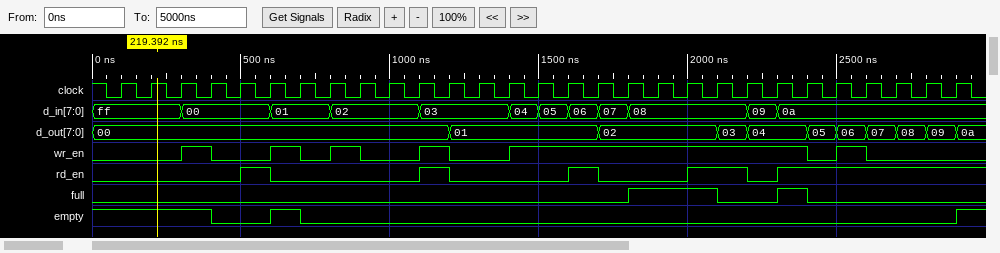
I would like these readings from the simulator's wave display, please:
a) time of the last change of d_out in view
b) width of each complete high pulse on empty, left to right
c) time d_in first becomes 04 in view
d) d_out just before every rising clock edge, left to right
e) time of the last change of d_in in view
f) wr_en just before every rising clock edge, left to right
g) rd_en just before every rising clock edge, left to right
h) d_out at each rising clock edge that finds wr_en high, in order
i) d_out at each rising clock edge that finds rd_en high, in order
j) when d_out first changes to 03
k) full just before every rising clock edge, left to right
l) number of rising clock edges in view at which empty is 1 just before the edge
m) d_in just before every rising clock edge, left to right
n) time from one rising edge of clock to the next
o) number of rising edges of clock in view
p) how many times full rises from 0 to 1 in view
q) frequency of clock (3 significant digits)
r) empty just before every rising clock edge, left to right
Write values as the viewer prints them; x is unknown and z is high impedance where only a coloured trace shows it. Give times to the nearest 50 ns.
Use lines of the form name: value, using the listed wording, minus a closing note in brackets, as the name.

time of the last change of d_out in view: 2900 ns
width of each complete high pulse on empty, left to right: 100 ns
time d_in first becomes 04 in view: 1400 ns
d_out just before every rising clock edge, left to right: 00, 00, 00, 00, 00, 00, 00, 00, 00, 00, 00, 00, 01, 01, 01, 01, 01, 02, 02, 02, 02, 03, 04, 04, 05, 06, 07, 08, 09
time of the last change of d_in in view: 2300 ns
wr_en just before every rising clock edge, left to right: 0 0 0 1 0 0 1 0 1 0 0 1 0 0 1 1 1 1 1 1 1 1 1 1 0 1 0 0 0
rd_en just before every rising clock edge, left to right: 0 0 0 0 0 1 0 0 0 0 0 1 0 0 0 0 1 0 0 0 1 1 0 1 1 1 1 1 1
d_out at each rising clock edge that finds wr_en high, in order: 00, 00, 00, 00, 01, 01, 01, 02, 02, 02, 02, 03, 04, 04, 06
d_out at each rising clock edge that finds rd_en high, in order: 00, 00, 01, 02, 03, 04, 05, 06, 07, 08, 09
when d_out first changes to 03: 2100 ns
full just before every rising clock edge, left to right: 0 0 0 0 0 0 0 0 0 0 0 0 0 0 0 0 0 0 1 1 1 0 0 1 0 0 0 0 0
number of rising clock edges in view at which empty is 1 just before the edge: 5
d_in just before every rising clock edge, left to right: ff, ff, ff, 00, 00, 00, 01, 01, 02, 02, 02, 03, 03, 03, 04, 05, 06, 07, 08, 08, 08, 08, 09, 0a, 0a, 0a, 0a, 0a, 0a
time from one rising edge of clock to the next: 100 ns
number of rising edges of clock in view: 29
how many times full rises from 0 to 1 in view: 2
frequency of clock: 10.0 MHz
empty just before every rising clock edge, left to right: 1 1 1 1 0 0 1 0 0 0 0 0 0 0 0 0 0 0 0 0 0 0 0 0 0 0 0 0 0
